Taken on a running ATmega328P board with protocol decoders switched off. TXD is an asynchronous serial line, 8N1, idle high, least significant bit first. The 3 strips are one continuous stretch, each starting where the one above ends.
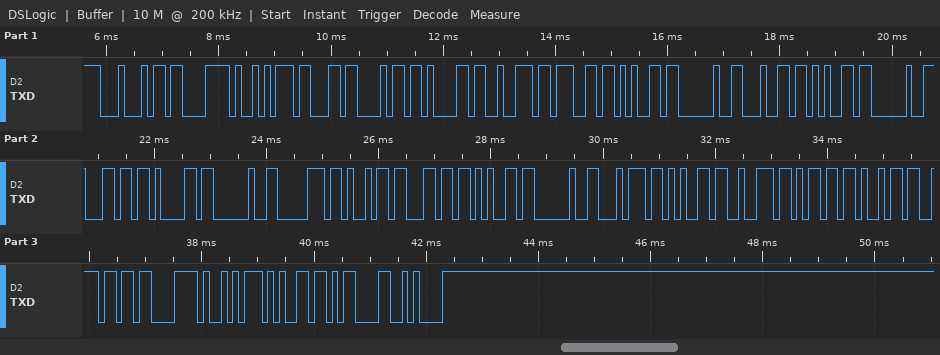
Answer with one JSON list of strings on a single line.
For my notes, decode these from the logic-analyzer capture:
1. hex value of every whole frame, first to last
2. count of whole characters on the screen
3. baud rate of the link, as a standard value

["44 C3 A9 63 68 61 72 67 65 20 64 65 20 6C 61 20 70 69 6C 65 20 74 65 72 6D 69 6E C3 A9 65 0D 0A", "32", "9600 baud"]
